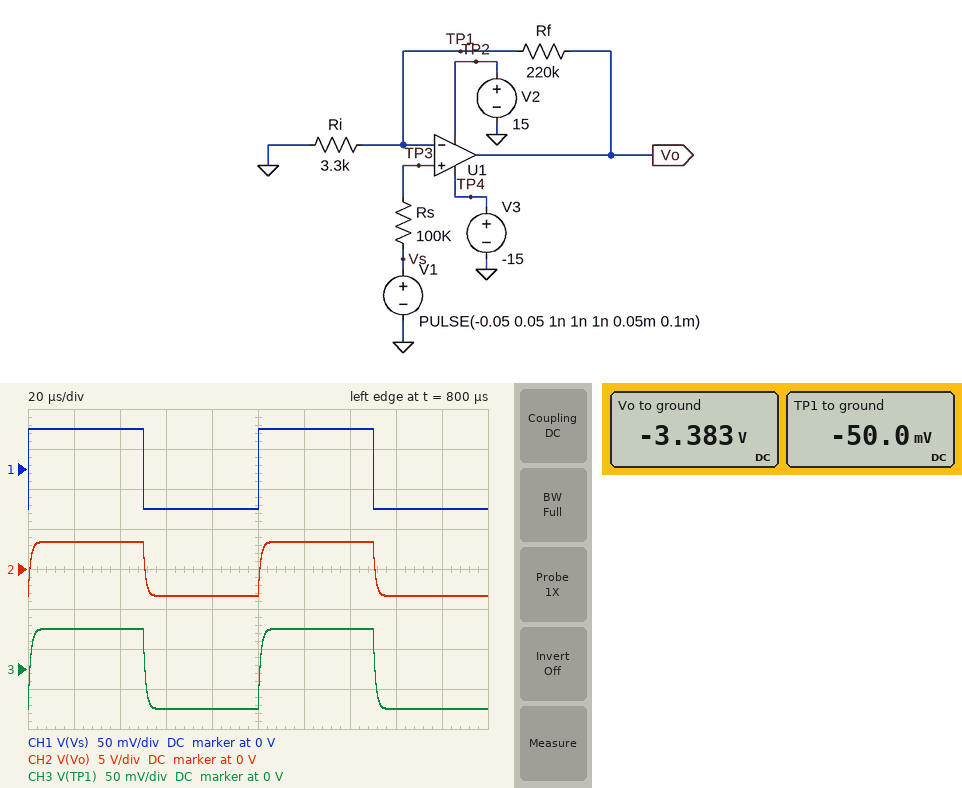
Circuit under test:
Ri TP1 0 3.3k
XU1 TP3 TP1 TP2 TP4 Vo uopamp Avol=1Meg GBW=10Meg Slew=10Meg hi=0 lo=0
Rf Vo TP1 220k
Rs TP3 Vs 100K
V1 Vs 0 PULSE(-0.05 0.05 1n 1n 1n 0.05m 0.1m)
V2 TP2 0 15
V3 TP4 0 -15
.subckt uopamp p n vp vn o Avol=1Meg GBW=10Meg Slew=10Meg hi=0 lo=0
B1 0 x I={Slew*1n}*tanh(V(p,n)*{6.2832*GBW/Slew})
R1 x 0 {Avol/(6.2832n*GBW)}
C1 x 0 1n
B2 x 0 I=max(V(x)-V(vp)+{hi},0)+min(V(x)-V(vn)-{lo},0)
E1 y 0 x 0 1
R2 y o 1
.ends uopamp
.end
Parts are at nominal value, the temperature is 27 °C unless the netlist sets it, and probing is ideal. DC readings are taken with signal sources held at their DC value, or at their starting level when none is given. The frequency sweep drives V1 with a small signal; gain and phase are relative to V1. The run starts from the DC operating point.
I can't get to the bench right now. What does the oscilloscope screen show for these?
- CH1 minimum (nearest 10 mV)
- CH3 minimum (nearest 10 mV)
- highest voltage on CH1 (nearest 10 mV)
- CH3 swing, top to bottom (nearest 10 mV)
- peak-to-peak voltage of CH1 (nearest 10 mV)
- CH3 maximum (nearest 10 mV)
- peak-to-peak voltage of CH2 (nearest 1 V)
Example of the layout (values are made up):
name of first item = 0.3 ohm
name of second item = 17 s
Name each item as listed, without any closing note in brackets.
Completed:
CH1 minimum = -50 mV
CH3 minimum = -50 mV
highest voltage on CH1 = 50 mV
CH3 swing, top to bottom = 100 mV
peak-to-peak voltage of CH1 = 100 mV
CH3 maximum = 50 mV
peak-to-peak voltage of CH2 = 7 V
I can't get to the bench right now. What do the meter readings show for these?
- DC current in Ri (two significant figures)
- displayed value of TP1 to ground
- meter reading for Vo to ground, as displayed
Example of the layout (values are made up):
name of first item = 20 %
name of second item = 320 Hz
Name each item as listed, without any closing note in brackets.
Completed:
DC current in Ri = 15 µA
displayed value of TP1 to ground = -50.0 mV
meter reading for Vo to ground, as displayed = -3.383 V
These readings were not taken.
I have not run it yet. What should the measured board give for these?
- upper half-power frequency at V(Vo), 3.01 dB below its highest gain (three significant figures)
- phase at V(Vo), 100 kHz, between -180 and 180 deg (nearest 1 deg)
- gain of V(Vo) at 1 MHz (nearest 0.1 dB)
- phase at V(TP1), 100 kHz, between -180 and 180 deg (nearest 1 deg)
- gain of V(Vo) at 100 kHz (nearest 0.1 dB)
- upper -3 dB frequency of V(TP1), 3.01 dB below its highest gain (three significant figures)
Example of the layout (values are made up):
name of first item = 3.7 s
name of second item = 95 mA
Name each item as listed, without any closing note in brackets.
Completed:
upper half-power frequency at V(Vo), 3.01 dB below its highest gain = 148 kHz
phase at V(Vo), 100 kHz, between -180 and 180 deg = -34 deg
gain of V(Vo) at 1 MHz = 19.9 dB
phase at V(TP1), 100 kHz, between -180 and 180 deg = -34 deg
gain of V(Vo) at 100 kHz = 35.0 dB
upper -3 dB frequency of V(TP1), 3.01 dB below its highest gain = 148 kHz
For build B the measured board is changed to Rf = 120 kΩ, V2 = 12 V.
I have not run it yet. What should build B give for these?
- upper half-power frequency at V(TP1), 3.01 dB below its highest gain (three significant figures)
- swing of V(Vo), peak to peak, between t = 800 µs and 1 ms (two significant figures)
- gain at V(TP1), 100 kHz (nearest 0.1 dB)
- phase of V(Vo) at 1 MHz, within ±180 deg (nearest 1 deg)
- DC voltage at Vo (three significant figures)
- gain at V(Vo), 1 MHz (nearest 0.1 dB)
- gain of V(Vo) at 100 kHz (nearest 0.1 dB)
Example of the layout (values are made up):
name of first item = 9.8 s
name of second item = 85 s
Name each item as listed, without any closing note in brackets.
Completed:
upper half-power frequency at V(TP1), 3.01 dB below its highest gain = 268 kHz
swing of V(Vo), peak to peak, between t = 800 µs and 1 ms = 3.7 V
gain at V(TP1), 100 kHz = -0.6 dB
phase of V(Vo) at 1 MHz, within ±180 deg = -75 deg
DC voltage at Vo = -1.87 V
gain at V(Vo), 1 MHz = 19.7 dB
gain of V(Vo) at 100 kHz = 30.9 dB
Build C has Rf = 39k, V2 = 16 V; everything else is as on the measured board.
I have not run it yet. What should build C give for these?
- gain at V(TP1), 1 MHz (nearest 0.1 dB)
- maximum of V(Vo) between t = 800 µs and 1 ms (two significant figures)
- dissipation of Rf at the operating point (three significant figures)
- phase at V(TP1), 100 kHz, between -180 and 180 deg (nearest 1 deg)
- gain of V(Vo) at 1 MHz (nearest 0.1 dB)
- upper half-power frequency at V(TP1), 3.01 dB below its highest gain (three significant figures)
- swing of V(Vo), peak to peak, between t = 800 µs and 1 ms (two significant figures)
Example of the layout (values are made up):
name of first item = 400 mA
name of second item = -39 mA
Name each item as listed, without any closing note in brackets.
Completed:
gain at V(TP1), 1 MHz = -4.2 dB
maximum of V(Vo) between t = 800 µs and 1 ms = 640 mV
dissipation of Rf at the operating point = 8.95 µW
phase at V(TP1), 100 kHz, between -180 and 180 deg = -7 deg
gain of V(Vo) at 1 MHz = 17.9 dB
upper half-power frequency at V(TP1), 3.01 dB below its highest gain = 780 kHz
swing of V(Vo), peak to peak, between t = 800 µs and 1 ms = 1.3 V
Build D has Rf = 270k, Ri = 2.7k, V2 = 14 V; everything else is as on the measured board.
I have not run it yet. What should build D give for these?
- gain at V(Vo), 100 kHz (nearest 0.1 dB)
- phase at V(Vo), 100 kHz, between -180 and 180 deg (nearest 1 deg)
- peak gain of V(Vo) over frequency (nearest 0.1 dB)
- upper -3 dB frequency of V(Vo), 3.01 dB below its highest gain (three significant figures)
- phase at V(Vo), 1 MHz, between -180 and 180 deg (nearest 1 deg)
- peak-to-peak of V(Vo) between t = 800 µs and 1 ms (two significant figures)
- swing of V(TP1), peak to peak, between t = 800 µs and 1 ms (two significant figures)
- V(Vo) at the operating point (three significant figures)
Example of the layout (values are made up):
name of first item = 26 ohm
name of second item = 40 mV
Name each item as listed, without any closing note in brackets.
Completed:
gain at V(Vo), 100 kHz = 37.0 dB
phase at V(Vo), 100 kHz, between -180 and 180 deg = -45 deg
peak gain of V(Vo) over frequency = 40.1 dB
upper -3 dB frequency of V(Vo), 3.01 dB below its highest gain = 99.0 kHz
phase at V(Vo), 1 MHz, between -180 and 180 deg = -84 deg
peak-to-peak of V(Vo) between t = 800 µs and 1 ms = 10 V
swing of V(TP1), peak to peak, between t = 800 µs and 1 ms = 100 mV
V(Vo) at the operating point = -5.05 V
